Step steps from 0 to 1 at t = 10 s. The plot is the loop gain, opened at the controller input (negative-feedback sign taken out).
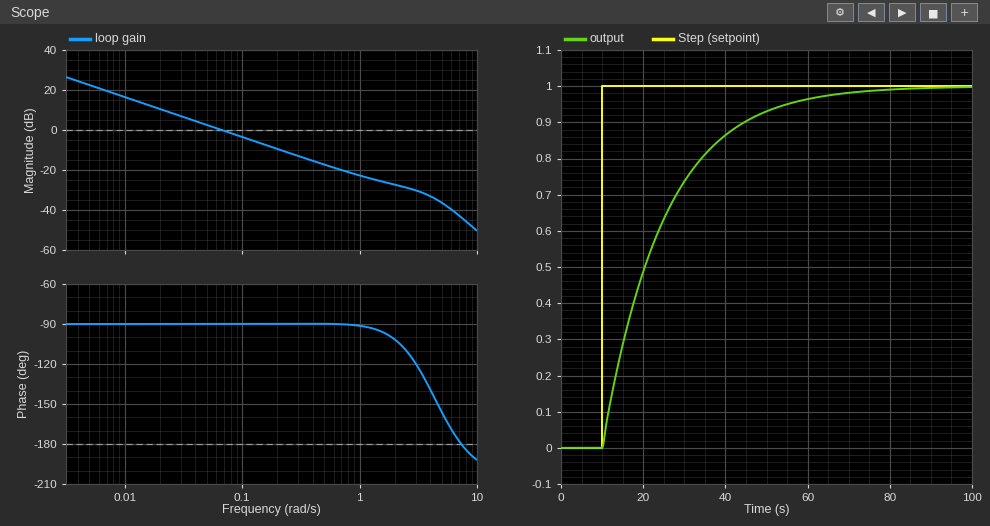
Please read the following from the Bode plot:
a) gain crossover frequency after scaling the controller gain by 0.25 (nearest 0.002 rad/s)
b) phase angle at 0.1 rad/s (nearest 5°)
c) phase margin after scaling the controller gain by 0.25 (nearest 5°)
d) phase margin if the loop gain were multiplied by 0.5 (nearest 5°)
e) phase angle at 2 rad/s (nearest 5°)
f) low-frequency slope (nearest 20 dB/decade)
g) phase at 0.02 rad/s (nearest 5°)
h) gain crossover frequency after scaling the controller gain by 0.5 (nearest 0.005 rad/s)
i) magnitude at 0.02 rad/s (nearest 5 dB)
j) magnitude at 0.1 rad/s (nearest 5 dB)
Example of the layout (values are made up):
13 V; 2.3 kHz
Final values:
0.016 rad/s; -90°; 90°; 90°; -100°; -20 dB/decade; -90°; 0.035 rad/s; 10 dB; -5 dB
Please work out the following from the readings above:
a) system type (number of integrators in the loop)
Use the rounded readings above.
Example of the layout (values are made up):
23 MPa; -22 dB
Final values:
1
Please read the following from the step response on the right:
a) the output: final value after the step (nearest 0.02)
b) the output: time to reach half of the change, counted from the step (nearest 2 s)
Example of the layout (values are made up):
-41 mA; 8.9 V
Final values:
1.00; 10 s
